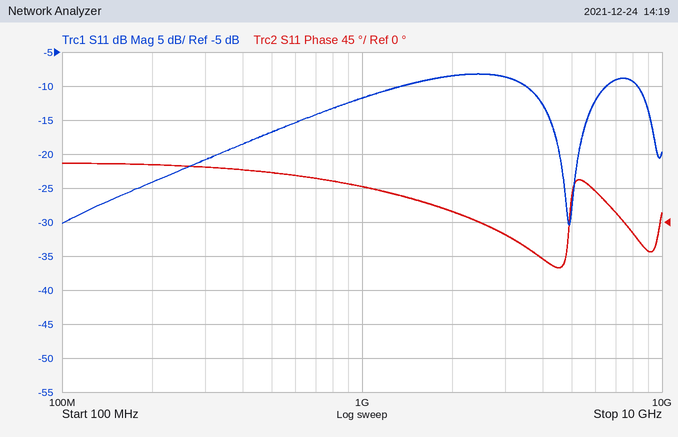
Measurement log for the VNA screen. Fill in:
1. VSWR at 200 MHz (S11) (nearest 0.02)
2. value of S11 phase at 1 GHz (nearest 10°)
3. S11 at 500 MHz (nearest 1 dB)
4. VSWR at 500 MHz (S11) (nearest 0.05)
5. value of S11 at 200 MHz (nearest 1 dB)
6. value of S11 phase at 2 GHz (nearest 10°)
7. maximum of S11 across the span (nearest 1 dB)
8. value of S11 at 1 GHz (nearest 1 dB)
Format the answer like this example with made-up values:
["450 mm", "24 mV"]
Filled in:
["1.14", "50°", "-17 dB", "1.35", "-24 dB", "10°", "-8 dB", "-12 dB"]
